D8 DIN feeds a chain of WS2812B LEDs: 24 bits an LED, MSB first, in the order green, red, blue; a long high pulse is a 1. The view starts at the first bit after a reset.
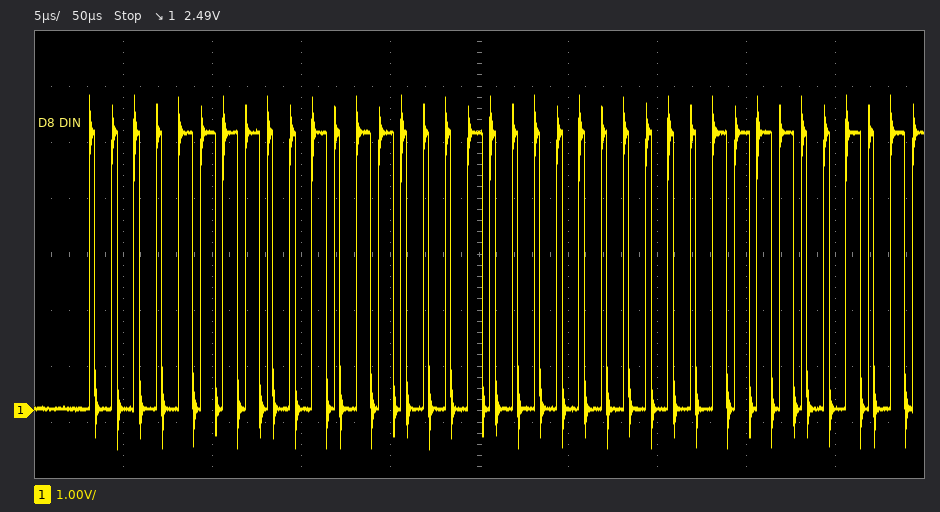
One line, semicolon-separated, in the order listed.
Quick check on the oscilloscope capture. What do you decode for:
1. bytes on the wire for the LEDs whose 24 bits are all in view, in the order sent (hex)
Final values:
0F 2C 40
